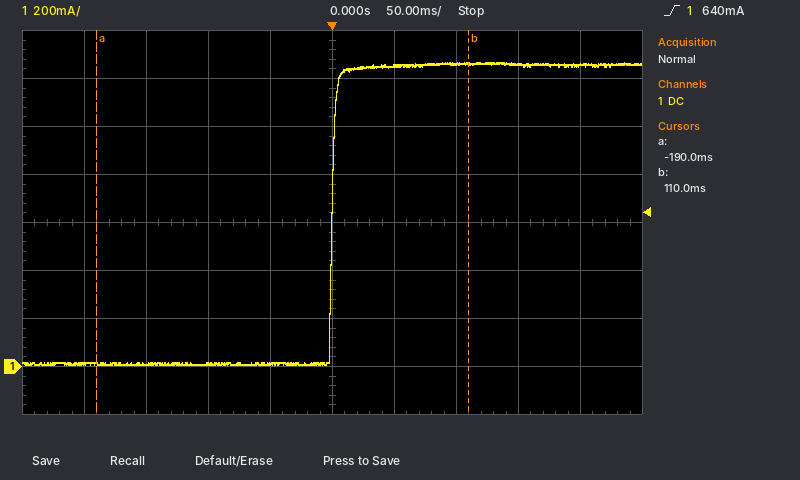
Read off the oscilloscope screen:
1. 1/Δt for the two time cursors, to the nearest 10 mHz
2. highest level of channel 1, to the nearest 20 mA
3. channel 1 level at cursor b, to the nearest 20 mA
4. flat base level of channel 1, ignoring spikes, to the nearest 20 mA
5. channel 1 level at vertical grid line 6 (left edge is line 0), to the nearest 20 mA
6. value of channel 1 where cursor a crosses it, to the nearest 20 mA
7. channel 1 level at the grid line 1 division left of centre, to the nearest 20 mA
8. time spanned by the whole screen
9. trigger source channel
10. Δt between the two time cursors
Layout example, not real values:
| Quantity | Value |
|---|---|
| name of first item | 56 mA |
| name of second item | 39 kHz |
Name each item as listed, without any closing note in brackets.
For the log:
| Quantity | Value |
|---|---|
| 1/Δt for the two time cursors, to the nearest 10 mHz | 3.33 Hz |
| highest level of channel 1, to the nearest 20 mA | 1.26 A |
| channel 1 level at cursor b, to the nearest 20 mA | 1.26 A |
| flat base level of channel 1, ignoring spikes, to the nearest 20 mA | 20 mA |
| channel 1 level at vertical grid line 6 (left edge is line 0), to the nearest 20 mA | 1.26 A |
| value of channel 1 where cursor a crosses it, to the nearest 20 mA | 20 mA |
| channel 1 level at the grid line 1 division left of centre, to the nearest 20 mA | 20 mA |
| time spanned by the whole screen | 500 ms |
| trigger source channel | channel 1 |
| Δt between the two time cursors | 300 ms |
